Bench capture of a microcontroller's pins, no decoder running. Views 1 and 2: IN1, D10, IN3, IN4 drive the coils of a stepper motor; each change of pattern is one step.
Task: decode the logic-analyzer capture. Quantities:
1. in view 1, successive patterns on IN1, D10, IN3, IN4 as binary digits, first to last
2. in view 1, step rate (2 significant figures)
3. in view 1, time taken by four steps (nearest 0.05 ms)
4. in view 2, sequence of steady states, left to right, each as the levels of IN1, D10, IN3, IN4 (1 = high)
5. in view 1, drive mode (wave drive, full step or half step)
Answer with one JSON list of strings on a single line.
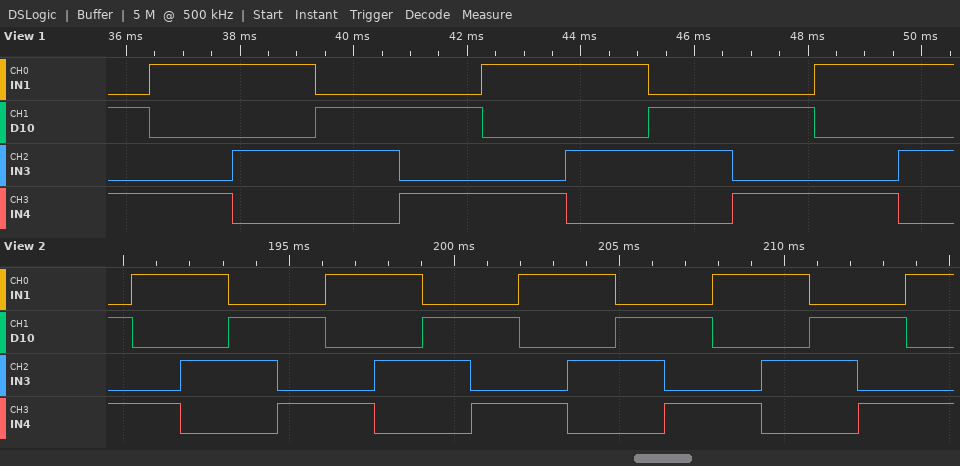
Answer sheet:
["0101 1001 1010 0110 0101 1001 1010 0110 0101 1001 1010", "680 steps/s", "5.85 ms", "0101 1001 1010 0110 0101 1001 1010 0110 0101 1001 1010 0110 0101 1001 1010 0110 0101 1001", "full step"]
